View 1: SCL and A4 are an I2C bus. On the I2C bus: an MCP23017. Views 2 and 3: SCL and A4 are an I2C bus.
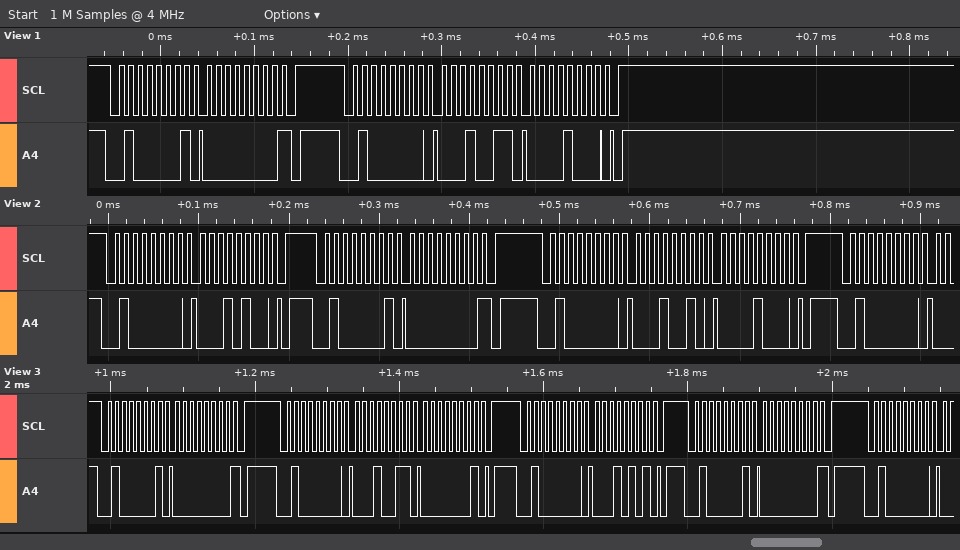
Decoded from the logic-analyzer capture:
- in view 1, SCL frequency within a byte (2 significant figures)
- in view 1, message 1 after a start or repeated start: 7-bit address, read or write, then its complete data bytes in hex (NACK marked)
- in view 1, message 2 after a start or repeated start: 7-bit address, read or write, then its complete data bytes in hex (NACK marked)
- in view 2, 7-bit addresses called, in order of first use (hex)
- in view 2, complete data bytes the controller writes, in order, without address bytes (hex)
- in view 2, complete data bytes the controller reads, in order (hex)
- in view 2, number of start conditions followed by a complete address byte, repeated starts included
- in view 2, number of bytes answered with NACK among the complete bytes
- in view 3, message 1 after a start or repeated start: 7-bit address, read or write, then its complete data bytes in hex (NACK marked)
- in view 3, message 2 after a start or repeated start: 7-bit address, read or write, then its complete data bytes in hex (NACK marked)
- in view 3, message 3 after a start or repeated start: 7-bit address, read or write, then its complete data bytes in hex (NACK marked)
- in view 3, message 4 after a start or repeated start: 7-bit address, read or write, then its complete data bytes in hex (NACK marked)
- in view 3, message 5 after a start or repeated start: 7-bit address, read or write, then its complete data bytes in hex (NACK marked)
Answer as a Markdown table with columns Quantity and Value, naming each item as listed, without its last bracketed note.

| Quantity | Value |
|---|---|
| in view 1, SCL frequency within a byte | 100 kHz |
| in view 1, message 1 after a start or repeated start: 7-bit address, read or write, then its complete data bytes in hex | 0x20 read: 00 NACK |
| in view 1, message 2 after a start or repeated start: 7-bit address, read or write, then its complete data bytes in hex | 0x20 write: 13 08 |
| in view 2, 7-bit addresses called, in order of first use | 0x20 |
| in view 2, complete data bytes the controller writes, in order, without address bytes | 14 12 08 |
| in view 2, complete data bytes the controller reads, in order | 00 |
| in view 2, number of start conditions followed by a complete address byte, repeated starts included | 4 |
| in view 2, number of bytes answered with NACK among the complete bytes | 1 |
| in view 3, message 1 after a start or repeated start: 7-bit address, read or write, then its complete data bytes in hex | 0x20 read: 00 NACK |
| in view 3, message 2 after a start or repeated start: 7-bit address, read or write, then its complete data bytes in hex | 0x20 write: 13 01 |
| in view 3, message 3 after a start or repeated start: 7-bit address, read or write, then its complete data bytes in hex | 0x20 write: 15 |
| in view 3, message 4 after a start or repeated start: 7-bit address, read or write, then its complete data bytes in hex | 0x20 read: 00 NACK |
| in view 3, message 5 after a start or repeated start: 7-bit address, read or write, then its complete data bytes in hex | 0x20 write |
